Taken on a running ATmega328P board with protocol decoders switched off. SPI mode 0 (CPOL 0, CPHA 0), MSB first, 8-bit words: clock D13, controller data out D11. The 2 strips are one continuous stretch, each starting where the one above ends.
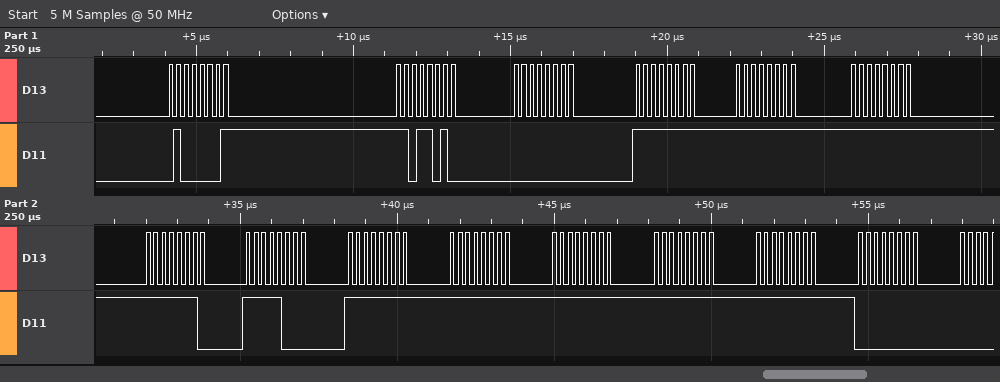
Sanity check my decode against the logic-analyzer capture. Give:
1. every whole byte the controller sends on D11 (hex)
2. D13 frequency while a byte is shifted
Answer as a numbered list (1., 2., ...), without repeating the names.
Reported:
1. 0x41 0xDA 0x00 0xFF 0xFF 0xFF 0xFE 0xF8 0xFF 0xFF 0xFF 0xFF 0xFF 0x00
2. 4 MHz
